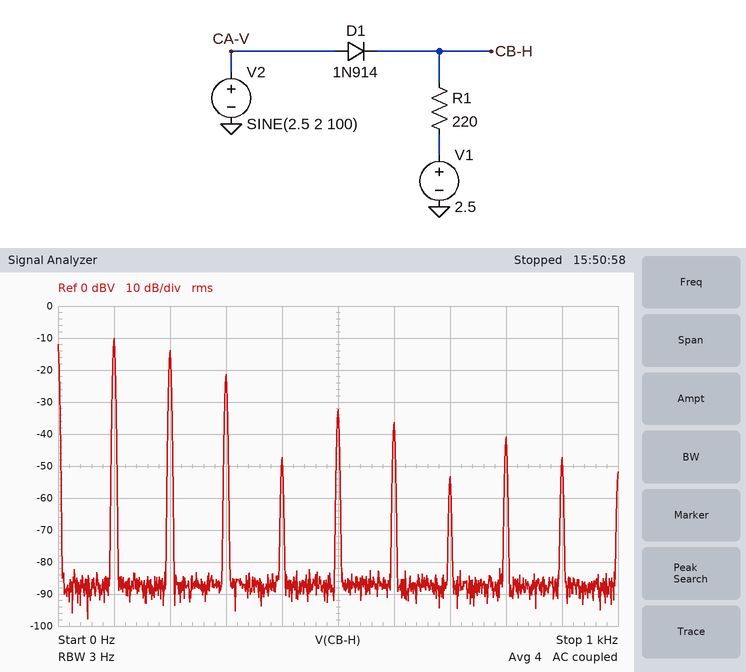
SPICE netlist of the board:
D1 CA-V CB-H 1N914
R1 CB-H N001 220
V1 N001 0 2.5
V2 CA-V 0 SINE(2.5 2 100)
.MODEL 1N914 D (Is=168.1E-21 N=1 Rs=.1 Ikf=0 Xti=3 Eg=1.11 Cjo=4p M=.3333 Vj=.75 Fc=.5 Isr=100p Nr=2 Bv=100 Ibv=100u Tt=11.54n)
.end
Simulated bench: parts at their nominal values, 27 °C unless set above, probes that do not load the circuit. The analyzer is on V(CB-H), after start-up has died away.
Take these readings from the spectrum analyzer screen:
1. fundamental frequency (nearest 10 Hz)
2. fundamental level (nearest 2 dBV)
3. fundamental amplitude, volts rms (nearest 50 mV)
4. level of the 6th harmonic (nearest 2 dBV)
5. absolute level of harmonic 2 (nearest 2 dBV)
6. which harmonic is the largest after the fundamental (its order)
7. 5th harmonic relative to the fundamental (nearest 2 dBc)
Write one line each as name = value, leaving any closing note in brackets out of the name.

fundamental frequency = 100 Hz
fundamental level = -10 dBV
fundamental amplitude, volts rms = 300 mV
level of the 6th harmonic = -36 dBV
absolute level of harmonic 2 = -14 dBV
which harmonic is the largest after the fundamental = 2
5th harmonic relative to the fundamental = -22 dBc
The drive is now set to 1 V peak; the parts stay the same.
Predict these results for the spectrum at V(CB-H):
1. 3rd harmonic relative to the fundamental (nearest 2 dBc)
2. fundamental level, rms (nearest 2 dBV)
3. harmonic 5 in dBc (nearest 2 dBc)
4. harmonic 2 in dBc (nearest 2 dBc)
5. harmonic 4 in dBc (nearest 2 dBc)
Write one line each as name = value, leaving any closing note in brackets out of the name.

3rd harmonic relative to the fundamental = -4 dBc
fundamental level, rms = -30 dBV
harmonic 5 in dBc = -14 dBc
harmonic 2 in dBc = -2 dBc
harmonic 4 in dBc = -8 dBc
